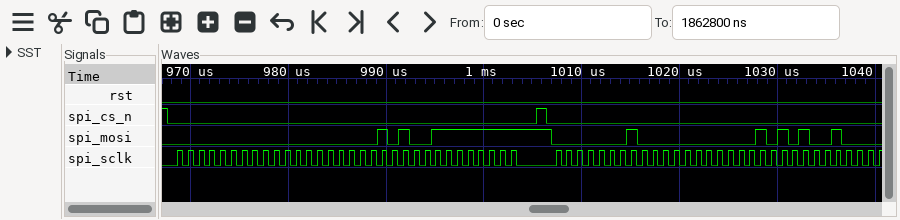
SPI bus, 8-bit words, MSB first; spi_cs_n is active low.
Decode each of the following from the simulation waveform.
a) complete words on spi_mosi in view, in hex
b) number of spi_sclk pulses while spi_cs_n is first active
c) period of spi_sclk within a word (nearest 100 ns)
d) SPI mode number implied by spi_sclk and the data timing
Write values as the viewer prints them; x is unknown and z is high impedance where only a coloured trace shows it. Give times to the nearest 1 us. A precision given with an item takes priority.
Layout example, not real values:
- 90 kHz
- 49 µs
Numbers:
- 00, 00, 14, FF, 01, 00, 15
- 32
- 1100 ns
- 0
